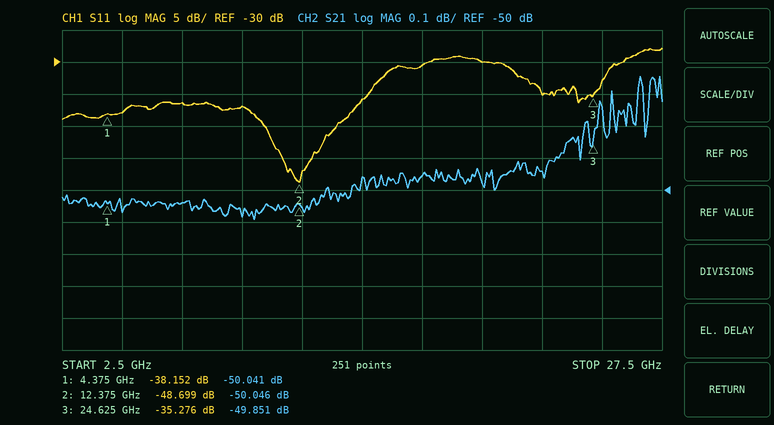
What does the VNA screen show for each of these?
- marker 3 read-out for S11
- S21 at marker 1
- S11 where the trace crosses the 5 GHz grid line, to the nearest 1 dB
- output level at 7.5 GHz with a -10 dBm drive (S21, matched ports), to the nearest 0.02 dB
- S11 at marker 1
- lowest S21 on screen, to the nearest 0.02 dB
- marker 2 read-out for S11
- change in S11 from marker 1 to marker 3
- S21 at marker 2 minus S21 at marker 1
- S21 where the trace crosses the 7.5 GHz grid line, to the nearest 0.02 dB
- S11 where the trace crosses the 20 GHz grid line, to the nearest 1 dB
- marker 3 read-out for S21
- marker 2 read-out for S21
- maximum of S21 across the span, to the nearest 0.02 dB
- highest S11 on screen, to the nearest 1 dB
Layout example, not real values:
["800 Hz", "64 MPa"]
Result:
["-35.276 dB", "-50.041 dB", "-38 dB", "-60.04 dBm", "-38.152 dB", "-50.10 dB", "-48.699 dB", "2.876 dB", "-0.005 dB", "-50.04 dB", "-30 dB", "-49.851 dB", "-50.046 dB", "-49.64 dB", "-28 dB"]
